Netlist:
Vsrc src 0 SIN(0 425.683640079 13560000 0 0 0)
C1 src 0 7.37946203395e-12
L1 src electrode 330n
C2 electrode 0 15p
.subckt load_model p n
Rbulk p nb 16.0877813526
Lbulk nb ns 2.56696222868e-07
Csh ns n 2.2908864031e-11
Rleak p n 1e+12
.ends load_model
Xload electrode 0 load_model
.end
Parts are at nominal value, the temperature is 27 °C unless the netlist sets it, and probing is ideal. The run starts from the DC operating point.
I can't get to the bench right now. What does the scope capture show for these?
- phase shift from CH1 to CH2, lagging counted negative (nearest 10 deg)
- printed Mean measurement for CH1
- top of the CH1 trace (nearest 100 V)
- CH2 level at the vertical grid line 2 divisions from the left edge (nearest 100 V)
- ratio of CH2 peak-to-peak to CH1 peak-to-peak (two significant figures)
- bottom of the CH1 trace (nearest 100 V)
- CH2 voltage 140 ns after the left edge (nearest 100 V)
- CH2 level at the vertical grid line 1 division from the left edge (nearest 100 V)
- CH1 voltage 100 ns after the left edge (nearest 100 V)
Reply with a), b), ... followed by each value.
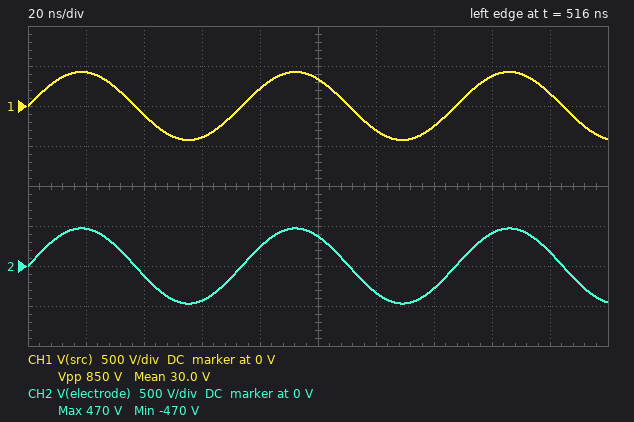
a) 0 deg
b) 30.0 V
c) 400 V
d) -100 V
e) 1.1
f) -400 V
g) -300 V
h) 500 V
i) 300 V
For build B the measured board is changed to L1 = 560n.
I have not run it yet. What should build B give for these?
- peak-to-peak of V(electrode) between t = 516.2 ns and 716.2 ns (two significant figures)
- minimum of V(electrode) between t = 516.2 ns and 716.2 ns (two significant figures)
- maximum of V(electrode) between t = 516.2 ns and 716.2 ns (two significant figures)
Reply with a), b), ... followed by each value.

a) 1.0 kV
b) -510 V
c) 510 V
